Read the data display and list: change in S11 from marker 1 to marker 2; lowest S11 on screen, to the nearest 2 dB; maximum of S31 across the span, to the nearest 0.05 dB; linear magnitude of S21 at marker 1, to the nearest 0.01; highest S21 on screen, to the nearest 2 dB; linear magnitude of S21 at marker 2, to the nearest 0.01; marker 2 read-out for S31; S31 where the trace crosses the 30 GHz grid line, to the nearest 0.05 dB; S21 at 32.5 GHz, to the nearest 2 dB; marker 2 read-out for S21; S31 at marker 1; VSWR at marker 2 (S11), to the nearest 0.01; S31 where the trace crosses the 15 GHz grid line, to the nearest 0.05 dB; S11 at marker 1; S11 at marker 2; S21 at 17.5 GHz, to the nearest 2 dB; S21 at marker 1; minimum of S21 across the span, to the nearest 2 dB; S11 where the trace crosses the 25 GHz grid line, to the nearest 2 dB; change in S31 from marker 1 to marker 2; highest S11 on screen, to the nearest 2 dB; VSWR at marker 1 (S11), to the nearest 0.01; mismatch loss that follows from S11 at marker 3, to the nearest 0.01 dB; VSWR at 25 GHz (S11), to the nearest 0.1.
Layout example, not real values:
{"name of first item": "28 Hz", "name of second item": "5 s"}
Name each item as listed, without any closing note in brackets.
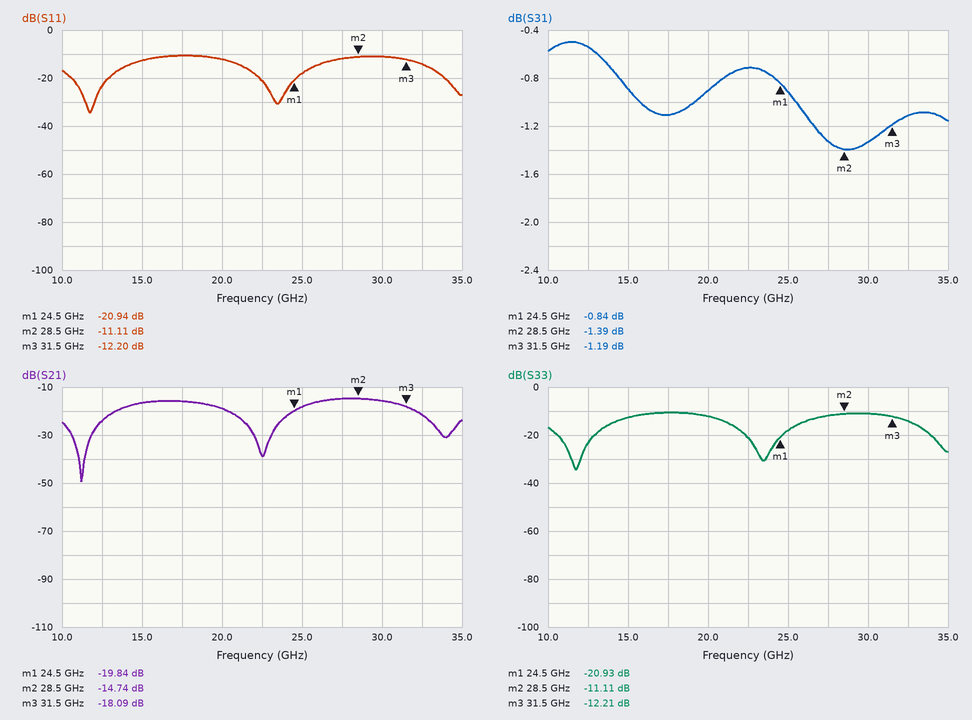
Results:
{"change in S11 from marker 1 to marker 2": "9.83 dB", "lowest S11 on screen, to the nearest 2 dB": "-34 dB", "maximum of S31 across the span, to the nearest 0.05 dB": "-0.50 dB", "linear magnitude of S21 at marker 1, to the nearest 0.01": "0.10", "highest S21 on screen, to the nearest 2 dB": "-14 dB", "linear magnitude of S21 at marker 2, to the nearest 0.01": "0.18", "marker 2 read-out for S31": "-1.39 dB", "S31 where the trace crosses the 30 GHz grid line, to the nearest 0.05 dB": "-1.35 dB", "S21 at 32.5 GHz, to the nearest 2 dB": "-22 dB", "marker 2 read-out for S21": "-14.74 dB", "S31 at marker 1": "-0.84 dB", "VSWR at marker 2 (S11), to the nearest 0.01": "1.77", "S31 where the trace crosses the 15 GHz grid line, to the nearest 0.05 dB": "-0.90 dB", "S11 at marker 1": "-20.94 dB", "S11 at marker 2": "-11.11 dB", "S21 at 17.5 GHz, to the nearest 2 dB": "-16 dB", "S21 at marker 1": "-19.84 dB", "minimum of S21 across the span, to the nearest 2 dB": "-50 dB", "S11 where the trace crosses the 25 GHz grid line, to the nearest 2 dB": "-18 dB", "change in S31 from marker 1 to marker 2": "-0.55 dB", "highest S11 on screen, to the nearest 2 dB": "-10 dB", "VSWR at marker 1 (S11), to the nearest 0.01": "1.20", "mismatch loss that follows from S11 at marker 3, to the nearest 0.01 dB": "0.27 dB", "VSWR at 25 GHz (S11), to the nearest 0.1": "1.3"}
